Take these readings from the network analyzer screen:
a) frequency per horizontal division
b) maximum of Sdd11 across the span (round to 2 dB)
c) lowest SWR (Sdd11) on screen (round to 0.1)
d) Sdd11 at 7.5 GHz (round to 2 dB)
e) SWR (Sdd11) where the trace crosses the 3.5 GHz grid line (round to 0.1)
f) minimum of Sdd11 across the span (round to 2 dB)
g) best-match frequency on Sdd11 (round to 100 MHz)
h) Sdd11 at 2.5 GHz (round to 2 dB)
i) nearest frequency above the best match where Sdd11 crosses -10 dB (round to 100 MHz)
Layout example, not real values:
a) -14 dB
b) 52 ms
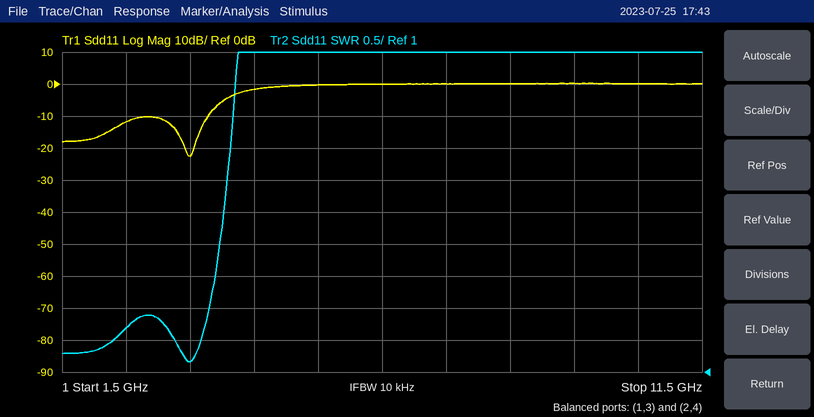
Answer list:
a) 1 GHz
b) 0 dB
c) 1.2
d) 0 dB
e) 1.2
f) -22 dB
g) 3.5 GHz
h) -12 dB
i) 3.8 GHz
